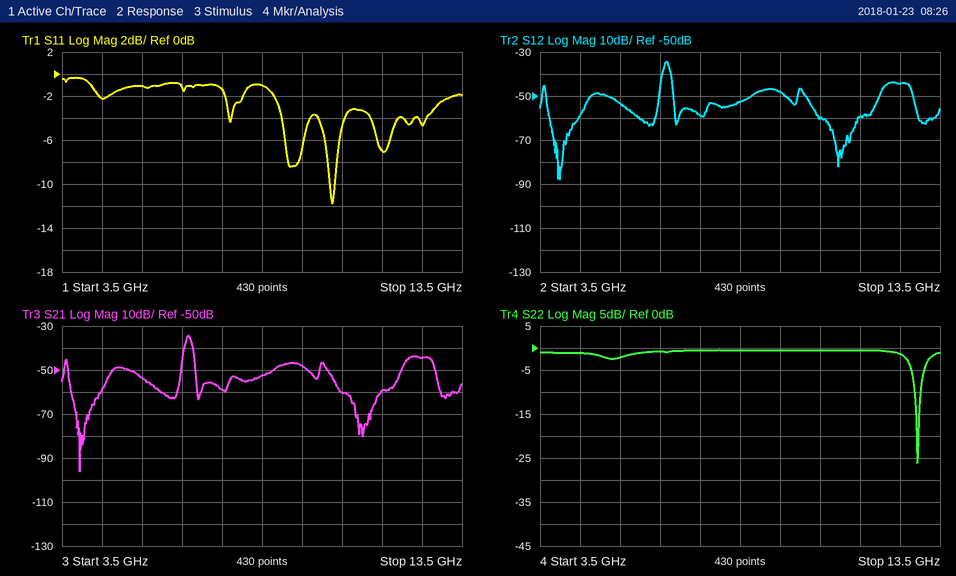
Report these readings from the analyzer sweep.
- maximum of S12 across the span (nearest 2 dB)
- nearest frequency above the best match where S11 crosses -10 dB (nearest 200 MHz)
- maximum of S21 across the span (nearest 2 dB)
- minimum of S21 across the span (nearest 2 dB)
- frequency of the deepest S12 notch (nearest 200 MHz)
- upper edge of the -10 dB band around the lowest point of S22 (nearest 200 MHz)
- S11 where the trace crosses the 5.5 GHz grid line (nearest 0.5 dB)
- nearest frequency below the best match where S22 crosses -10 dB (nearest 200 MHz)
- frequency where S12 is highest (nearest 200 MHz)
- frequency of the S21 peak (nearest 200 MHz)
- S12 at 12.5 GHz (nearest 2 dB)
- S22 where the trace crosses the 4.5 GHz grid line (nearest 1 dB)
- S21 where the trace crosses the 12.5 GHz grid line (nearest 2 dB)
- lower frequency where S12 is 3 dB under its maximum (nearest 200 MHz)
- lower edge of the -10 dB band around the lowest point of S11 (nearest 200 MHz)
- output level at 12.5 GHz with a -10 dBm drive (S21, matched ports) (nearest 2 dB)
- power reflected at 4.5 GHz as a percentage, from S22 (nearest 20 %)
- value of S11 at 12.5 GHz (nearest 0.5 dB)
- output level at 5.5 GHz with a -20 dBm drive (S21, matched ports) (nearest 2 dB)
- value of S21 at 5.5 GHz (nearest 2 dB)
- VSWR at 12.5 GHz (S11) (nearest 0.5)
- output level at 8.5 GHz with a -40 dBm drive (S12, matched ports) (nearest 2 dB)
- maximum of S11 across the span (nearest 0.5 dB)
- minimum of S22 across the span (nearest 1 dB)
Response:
-34 dB
10.4 GHz
-34 dB
-96 dB
4.0 GHz
13.0 GHz
-1.0 dB
12.8 GHz
6.6 GHz
6.6 GHz
-44 dB
-1 dB
-44 dB
6.6 GHz
10.2 GHz
-54 dBm
80 %
-4.5 dB
-74 dBm
-54 dB
4.0
-92 dBm
-0.5 dB
-26 dB
